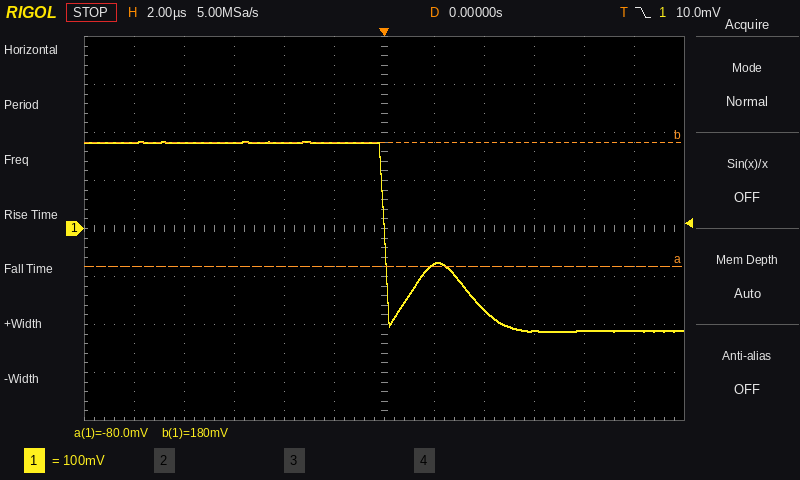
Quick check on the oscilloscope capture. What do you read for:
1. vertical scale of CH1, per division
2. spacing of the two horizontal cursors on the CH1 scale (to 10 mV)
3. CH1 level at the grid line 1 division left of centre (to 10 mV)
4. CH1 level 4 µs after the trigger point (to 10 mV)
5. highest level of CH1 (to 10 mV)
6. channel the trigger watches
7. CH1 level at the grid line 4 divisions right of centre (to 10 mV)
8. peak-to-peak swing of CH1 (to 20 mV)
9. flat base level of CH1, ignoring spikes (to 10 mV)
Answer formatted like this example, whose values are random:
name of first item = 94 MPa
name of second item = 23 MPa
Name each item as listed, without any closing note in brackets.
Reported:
vertical scale of CH1, per division = 100 mV
spacing of the two horizontal cursors on the CH1 scale = 260 mV
CH1 level at the grid line 1 division left of centre = 180 mV
CH1 level 4 µs after the trigger point = -170 mV
highest level of CH1 = 180 mV
channel the trigger watches = CH1
CH1 level at the grid line 4 divisions right of centre = -210 mV
peak-to-peak swing of CH1 = 400 mV
flat base level of CH1, ignoring spikes = -210 mV
